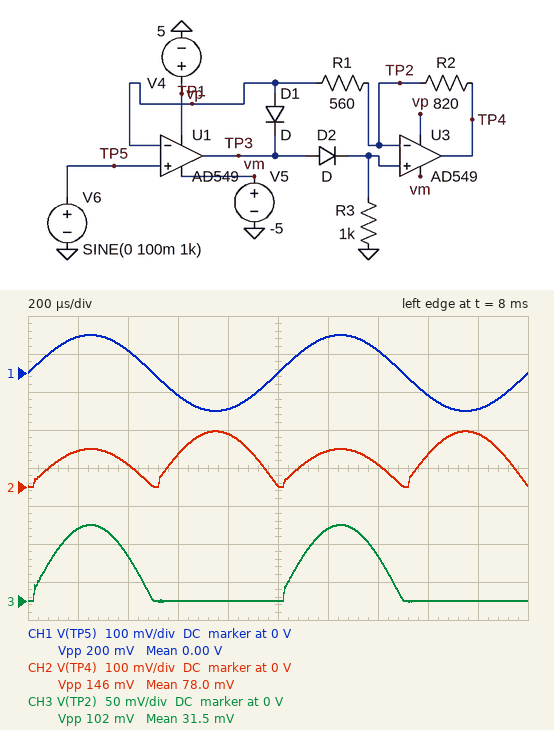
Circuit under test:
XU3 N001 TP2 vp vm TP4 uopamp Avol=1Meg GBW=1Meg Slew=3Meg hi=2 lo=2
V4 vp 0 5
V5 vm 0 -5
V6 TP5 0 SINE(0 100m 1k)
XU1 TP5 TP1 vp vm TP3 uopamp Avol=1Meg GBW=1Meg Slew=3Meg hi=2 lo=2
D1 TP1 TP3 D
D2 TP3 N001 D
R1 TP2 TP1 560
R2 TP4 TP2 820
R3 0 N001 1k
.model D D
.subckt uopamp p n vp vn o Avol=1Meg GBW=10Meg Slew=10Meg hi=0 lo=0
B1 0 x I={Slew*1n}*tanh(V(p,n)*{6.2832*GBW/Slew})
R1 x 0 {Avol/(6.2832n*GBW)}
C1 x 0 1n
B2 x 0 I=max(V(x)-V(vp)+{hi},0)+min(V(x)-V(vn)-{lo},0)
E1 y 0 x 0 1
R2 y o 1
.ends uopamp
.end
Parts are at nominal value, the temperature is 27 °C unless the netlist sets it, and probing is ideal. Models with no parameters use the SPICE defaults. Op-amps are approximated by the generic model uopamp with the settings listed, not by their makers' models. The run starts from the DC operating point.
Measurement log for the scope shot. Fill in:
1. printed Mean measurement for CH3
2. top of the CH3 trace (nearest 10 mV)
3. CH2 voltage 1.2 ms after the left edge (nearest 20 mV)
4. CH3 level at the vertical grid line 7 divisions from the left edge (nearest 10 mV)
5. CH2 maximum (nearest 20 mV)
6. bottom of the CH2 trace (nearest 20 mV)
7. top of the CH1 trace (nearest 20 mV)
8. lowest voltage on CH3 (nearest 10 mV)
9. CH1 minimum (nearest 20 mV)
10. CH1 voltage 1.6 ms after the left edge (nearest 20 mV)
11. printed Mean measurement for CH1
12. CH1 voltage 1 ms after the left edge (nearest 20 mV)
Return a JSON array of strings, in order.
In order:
["31.5 mV", "100 mV", "100 mV", "60 mV", "140 mV", "0 V", "100 mV", "0 V", "-100 mV", "-60 mV", "0.00 V", "0 V"]
